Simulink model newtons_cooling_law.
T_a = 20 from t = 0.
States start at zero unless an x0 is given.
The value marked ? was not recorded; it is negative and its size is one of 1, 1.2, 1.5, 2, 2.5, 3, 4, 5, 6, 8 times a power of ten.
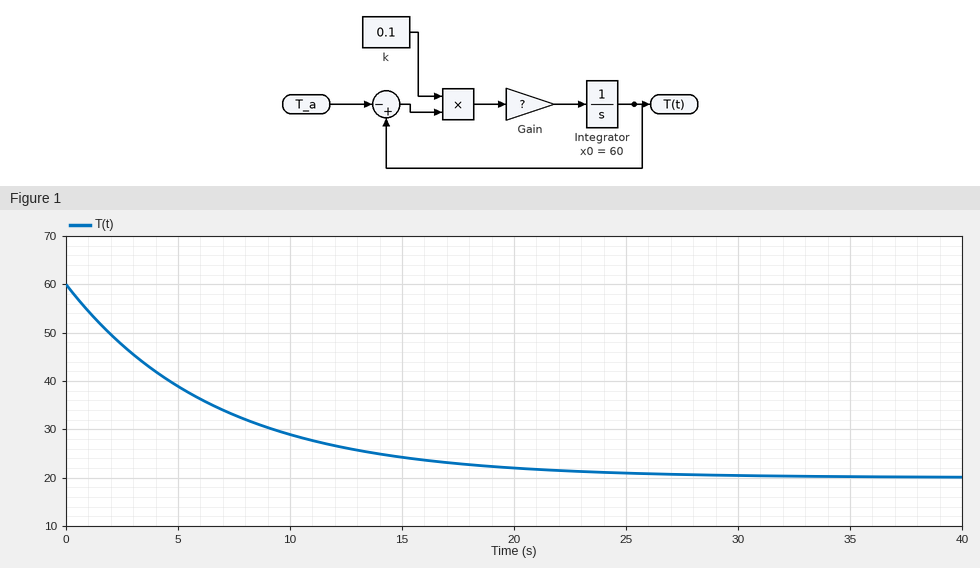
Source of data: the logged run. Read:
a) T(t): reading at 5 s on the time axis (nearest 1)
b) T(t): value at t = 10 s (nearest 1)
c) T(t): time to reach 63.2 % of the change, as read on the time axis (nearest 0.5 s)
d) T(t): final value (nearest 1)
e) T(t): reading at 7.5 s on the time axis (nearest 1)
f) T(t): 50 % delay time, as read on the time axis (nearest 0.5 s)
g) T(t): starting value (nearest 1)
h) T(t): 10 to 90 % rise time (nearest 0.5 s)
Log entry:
39
29
6.5 s
20
33
4.5 s
60
14.5 s
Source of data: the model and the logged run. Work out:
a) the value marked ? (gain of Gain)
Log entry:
-1.5
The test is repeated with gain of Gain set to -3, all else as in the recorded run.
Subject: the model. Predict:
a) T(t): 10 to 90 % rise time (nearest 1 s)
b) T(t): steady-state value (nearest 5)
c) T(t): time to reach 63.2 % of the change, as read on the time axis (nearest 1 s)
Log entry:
7 s
20
3 s
